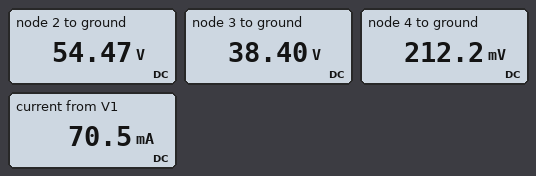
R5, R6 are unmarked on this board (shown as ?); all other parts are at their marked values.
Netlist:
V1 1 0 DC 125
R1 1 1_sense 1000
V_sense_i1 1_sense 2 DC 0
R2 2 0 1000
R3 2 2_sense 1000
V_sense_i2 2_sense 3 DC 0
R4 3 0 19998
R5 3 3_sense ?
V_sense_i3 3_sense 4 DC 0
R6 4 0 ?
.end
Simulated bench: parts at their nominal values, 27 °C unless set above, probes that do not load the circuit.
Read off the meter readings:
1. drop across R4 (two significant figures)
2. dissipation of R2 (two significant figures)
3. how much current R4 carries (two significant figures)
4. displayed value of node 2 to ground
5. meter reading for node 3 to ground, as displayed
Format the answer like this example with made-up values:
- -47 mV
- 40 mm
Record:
- 38 V
- 3.0 W
- 1.9 mA
- 54.47 V
- 38.40 V
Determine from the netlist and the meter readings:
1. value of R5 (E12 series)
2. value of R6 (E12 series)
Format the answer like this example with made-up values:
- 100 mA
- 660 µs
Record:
- 2.7 kΩ
- 15 Ω
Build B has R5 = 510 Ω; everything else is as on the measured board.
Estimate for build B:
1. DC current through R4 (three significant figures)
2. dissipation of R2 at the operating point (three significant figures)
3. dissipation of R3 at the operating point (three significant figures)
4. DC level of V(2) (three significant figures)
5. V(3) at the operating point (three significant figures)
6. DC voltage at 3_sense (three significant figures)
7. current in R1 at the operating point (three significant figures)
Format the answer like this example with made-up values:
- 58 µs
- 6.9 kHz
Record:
- 795 µA
- 2.21 W
- 965 mW
- 47.0 V
- 15.9 V
- 454 mV
- 78.0 mA
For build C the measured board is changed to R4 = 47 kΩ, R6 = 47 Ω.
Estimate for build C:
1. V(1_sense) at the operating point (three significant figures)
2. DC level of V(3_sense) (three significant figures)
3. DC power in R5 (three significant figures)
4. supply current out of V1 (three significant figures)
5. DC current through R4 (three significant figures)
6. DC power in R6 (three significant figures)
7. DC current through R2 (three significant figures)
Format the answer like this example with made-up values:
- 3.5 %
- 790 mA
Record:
- 54.9 V
- 678 mV
- 561 mW
- 70.1 mA
- 843 µA
- 9.77 mW
- 54.9 mA
